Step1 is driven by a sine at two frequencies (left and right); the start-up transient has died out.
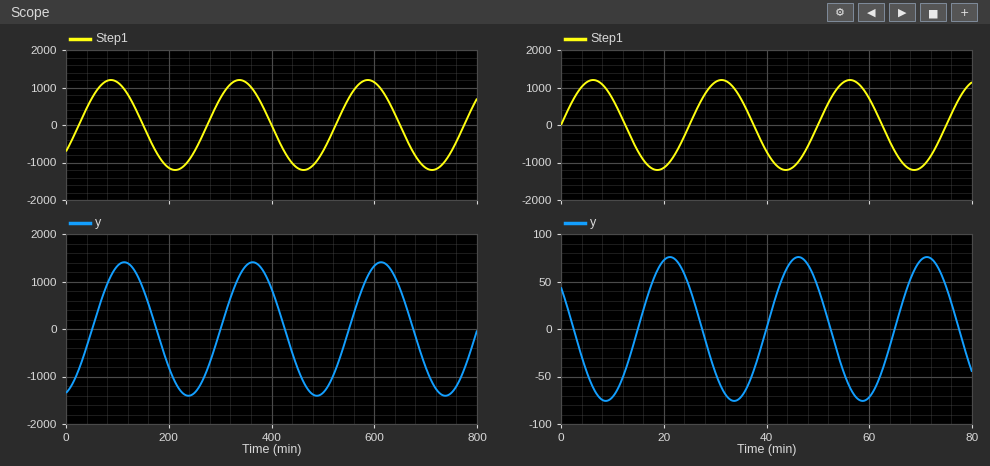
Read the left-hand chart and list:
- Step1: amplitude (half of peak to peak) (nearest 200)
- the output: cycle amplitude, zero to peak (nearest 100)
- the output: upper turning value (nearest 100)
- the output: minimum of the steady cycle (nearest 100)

1200
1400
1400
-1400
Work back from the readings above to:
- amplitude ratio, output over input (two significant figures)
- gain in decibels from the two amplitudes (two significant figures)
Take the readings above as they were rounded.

1.2
1.3 dB
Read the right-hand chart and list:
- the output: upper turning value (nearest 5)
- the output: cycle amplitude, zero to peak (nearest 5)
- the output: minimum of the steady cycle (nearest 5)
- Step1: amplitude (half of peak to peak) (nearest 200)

75
75
-75
1200
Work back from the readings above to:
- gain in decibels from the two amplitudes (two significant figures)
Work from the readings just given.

-24 dB
